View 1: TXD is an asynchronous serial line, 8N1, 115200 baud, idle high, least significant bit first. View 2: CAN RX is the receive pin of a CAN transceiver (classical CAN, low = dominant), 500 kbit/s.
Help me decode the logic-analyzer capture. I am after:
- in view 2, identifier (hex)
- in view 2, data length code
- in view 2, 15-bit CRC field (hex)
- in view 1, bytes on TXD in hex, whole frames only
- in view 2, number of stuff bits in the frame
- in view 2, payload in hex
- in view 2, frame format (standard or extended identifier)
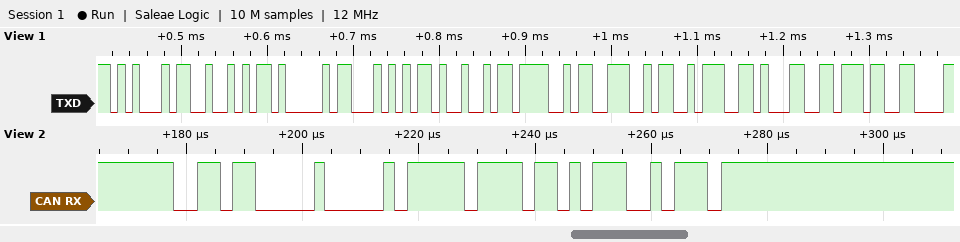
0x360
1
0x35CB
0x45 0x52 0x41 0x54 0x49 0x4F 0x4E 0x3A 0x31 0x37
3
FF
standard
